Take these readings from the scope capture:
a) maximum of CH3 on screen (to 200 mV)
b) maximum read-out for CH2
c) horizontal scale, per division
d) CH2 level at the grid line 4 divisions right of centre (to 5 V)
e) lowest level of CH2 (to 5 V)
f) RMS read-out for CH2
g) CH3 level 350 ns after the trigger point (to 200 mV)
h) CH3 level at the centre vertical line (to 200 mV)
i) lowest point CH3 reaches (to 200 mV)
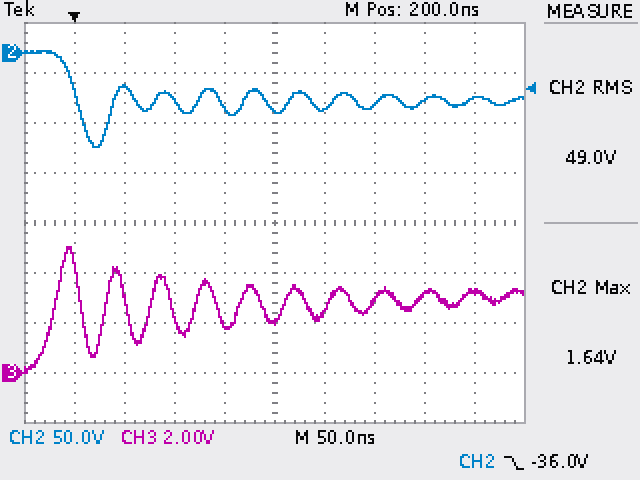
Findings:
5.0 V
1.64 V
50 ns
-45 V
-95 V
49.0 V
3.2 V
2.0 V
0.0 V
